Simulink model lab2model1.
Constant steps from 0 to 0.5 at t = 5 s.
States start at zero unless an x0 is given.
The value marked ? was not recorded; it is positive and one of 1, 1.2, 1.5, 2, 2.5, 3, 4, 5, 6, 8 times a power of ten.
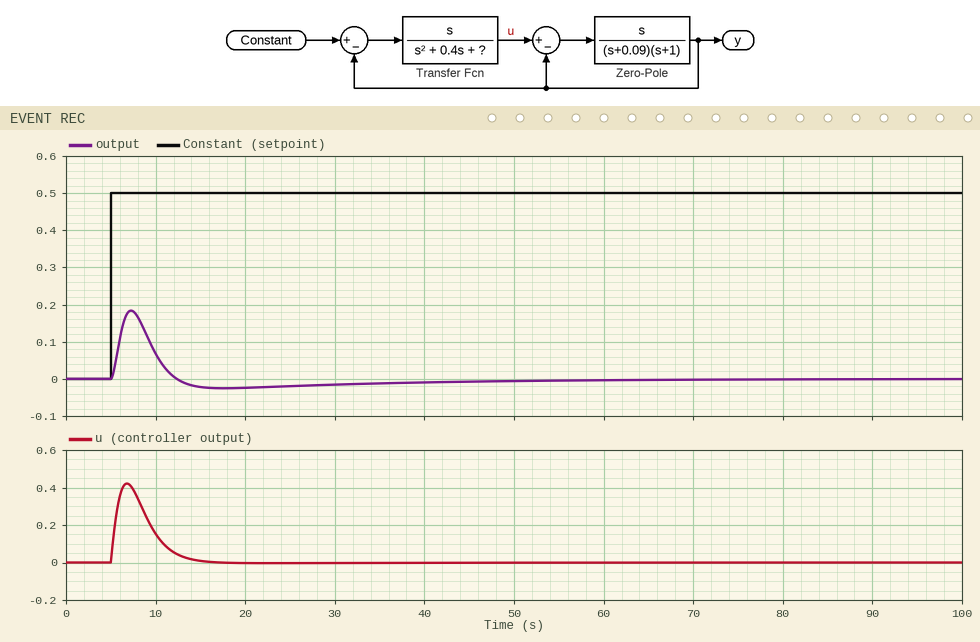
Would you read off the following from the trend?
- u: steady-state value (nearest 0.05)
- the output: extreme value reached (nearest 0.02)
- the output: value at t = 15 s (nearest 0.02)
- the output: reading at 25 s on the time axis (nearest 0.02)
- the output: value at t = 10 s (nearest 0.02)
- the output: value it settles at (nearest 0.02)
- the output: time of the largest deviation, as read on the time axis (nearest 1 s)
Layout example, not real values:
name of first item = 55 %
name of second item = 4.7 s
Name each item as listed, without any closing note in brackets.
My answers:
u: steady-state value = 0.00
the output: extreme value reached = 0.18
the output: value at t = 15 s = -0.02
the output: reading at 25 s on the time axis = -0.02
the output: value at t = 10 s = 0.06
the output: value it settles at = 0.00
the output: time of the largest deviation, as read on the time axis = 7 s
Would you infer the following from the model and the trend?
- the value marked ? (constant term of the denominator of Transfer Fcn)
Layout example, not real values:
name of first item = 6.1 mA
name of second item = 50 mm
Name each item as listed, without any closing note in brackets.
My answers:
the value marked ? = 0.3
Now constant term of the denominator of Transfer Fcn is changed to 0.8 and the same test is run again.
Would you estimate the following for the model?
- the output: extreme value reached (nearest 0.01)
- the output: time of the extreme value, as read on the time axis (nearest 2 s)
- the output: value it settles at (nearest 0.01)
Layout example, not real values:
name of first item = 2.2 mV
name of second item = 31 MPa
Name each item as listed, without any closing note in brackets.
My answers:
the output: extreme value reached = 0.14
the output: time of the extreme value, as read on the time axis = 6 s
the output: value it settles at = 0.00
